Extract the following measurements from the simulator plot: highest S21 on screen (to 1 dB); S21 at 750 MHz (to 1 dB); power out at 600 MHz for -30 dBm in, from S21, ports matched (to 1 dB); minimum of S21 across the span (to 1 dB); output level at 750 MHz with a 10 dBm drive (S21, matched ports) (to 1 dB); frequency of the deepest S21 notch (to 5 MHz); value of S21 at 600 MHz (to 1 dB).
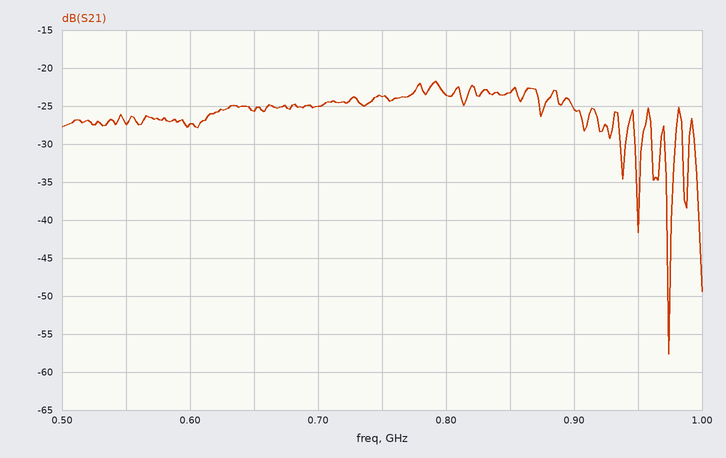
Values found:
-22 dB
-24 dB
-57 dBm
-58 dB
-14 dBm
975 MHz
-27 dB
